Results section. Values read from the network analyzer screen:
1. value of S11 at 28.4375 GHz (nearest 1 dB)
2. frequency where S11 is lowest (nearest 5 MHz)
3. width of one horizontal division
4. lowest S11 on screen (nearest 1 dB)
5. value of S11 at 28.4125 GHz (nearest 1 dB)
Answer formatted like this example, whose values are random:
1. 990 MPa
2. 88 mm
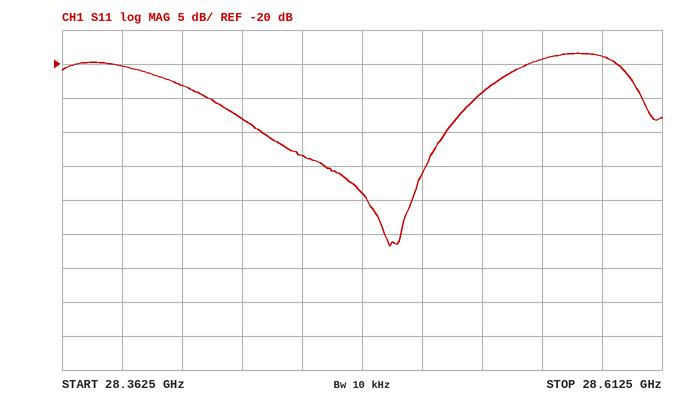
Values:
1. -28 dB
2. 28.500 GHz
3. 25 MHz
4. -47 dB
5. -23 dB
